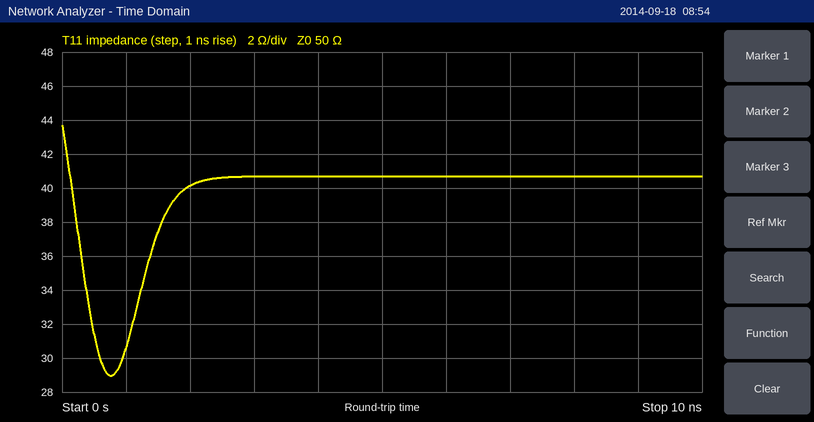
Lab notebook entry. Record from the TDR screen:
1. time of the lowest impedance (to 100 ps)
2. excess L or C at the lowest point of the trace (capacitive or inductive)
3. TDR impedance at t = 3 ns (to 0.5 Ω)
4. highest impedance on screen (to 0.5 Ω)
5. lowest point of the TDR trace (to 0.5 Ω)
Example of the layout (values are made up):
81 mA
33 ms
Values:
800 ps
capacitive
40.5 Ω
43.5 Ω
29.0 Ω
